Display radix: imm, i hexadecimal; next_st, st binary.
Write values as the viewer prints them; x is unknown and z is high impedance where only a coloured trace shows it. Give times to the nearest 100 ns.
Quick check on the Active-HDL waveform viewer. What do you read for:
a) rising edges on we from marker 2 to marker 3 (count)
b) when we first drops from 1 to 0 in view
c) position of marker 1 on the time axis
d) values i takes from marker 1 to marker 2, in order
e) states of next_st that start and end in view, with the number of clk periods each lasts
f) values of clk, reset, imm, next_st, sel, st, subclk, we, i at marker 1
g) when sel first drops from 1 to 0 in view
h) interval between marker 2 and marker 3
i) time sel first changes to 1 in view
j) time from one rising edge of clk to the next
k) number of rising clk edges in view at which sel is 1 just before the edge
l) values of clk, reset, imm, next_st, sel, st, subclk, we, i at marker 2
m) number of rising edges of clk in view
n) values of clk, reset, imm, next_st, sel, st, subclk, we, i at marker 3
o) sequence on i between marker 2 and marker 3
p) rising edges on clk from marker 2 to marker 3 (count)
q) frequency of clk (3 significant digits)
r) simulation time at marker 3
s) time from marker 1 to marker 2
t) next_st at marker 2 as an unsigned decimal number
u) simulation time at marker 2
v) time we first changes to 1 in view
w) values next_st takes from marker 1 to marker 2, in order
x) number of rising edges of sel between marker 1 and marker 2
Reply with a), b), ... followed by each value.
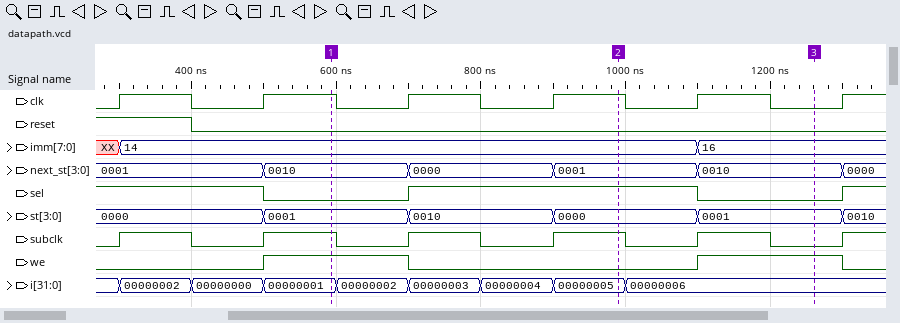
a) 1
b) 700 ns
c) 600 ns
d) 00000001, 00000002, 00000003, 00000004, 00000005
e) 0010: 1, 0000: 1, 0001: 1, 0010: 1
f) clk=1, reset=0, imm=14, next_st=0010, sel=0, st=0001, subclk=1, we=1, i=00000001
g) 500 ns
h) 300 ns
i) 700 ns
j) 200 ns
k) 4
l) clk=1, reset=0, imm=14, next_st=0001, sel=1, st=0000, subclk=1, we=0, i=00000005
m) 6
n) clk=0, reset=0, imm=16, next_st=0010, sel=0, st=0001, subclk=0, we=1, i=00000006
o) 00000005, 00000006
p) 1
q) 5.00 MHz
r) 1300 ns
s) 400 ns
t) 1
u) 1000 ns
v) 500 ns
w) 0010, 0000, 0001
x) 1
